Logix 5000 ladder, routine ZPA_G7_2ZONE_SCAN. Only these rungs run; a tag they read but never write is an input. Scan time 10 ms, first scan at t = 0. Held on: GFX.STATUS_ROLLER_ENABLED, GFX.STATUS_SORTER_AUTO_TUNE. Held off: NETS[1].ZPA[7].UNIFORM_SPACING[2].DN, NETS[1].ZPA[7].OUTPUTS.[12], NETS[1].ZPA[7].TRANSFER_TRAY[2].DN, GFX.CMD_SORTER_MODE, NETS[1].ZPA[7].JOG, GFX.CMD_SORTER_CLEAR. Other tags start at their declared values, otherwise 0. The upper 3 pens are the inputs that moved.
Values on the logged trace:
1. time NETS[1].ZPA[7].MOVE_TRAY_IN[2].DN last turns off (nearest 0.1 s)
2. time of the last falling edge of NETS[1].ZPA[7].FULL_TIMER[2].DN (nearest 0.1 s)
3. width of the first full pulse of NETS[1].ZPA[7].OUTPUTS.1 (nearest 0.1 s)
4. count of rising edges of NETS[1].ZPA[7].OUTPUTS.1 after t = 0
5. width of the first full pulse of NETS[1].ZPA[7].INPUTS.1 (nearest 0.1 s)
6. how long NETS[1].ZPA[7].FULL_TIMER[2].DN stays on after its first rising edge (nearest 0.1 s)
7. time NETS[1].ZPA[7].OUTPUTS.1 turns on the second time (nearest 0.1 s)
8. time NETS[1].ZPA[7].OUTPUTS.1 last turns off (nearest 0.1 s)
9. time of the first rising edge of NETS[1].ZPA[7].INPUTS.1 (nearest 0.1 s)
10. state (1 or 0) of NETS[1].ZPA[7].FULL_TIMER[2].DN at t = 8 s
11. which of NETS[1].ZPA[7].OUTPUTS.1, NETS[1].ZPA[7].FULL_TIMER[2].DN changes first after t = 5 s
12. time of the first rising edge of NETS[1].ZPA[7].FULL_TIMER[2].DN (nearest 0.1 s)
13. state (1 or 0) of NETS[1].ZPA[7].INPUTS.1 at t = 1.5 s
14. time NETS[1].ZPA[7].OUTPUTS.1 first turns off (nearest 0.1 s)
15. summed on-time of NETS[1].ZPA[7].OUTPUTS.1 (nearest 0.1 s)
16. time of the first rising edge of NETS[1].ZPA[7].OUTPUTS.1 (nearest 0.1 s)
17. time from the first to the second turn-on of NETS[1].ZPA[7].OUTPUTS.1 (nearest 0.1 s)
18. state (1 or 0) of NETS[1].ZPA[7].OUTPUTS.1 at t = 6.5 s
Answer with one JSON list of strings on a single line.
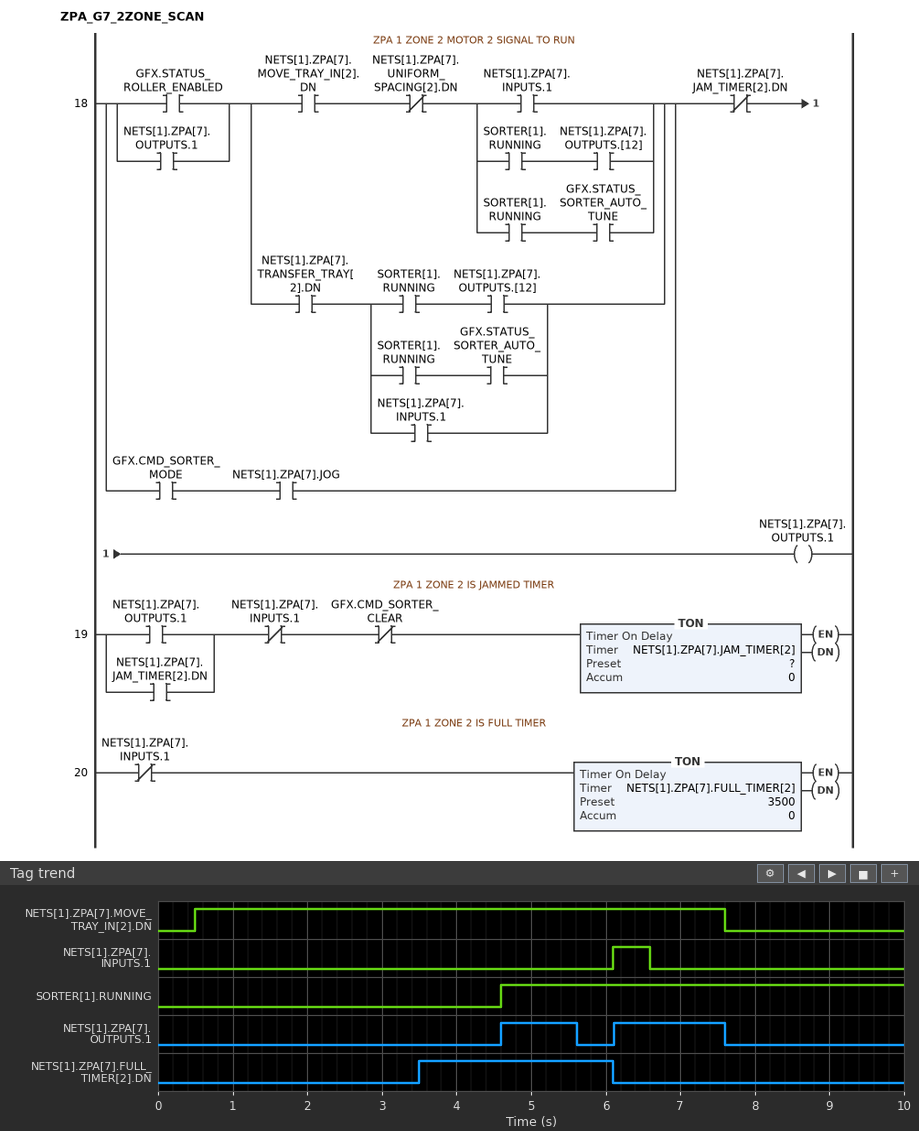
["7.6 s", "6.1 s", "1.0 s", "2", "0.5 s", "2.6 s", "6.1 s", "7.6 s", "6.1 s", "0", "NETS[1].ZPA[7].OUTPUTS.1", "3.5 s", "0", "5.6 s", "2.5 s", "4.6 s", "1.5 s", "1"]
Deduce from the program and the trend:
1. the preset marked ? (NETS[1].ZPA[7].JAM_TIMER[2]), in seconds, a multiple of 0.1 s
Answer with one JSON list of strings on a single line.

["1.0 s"]
